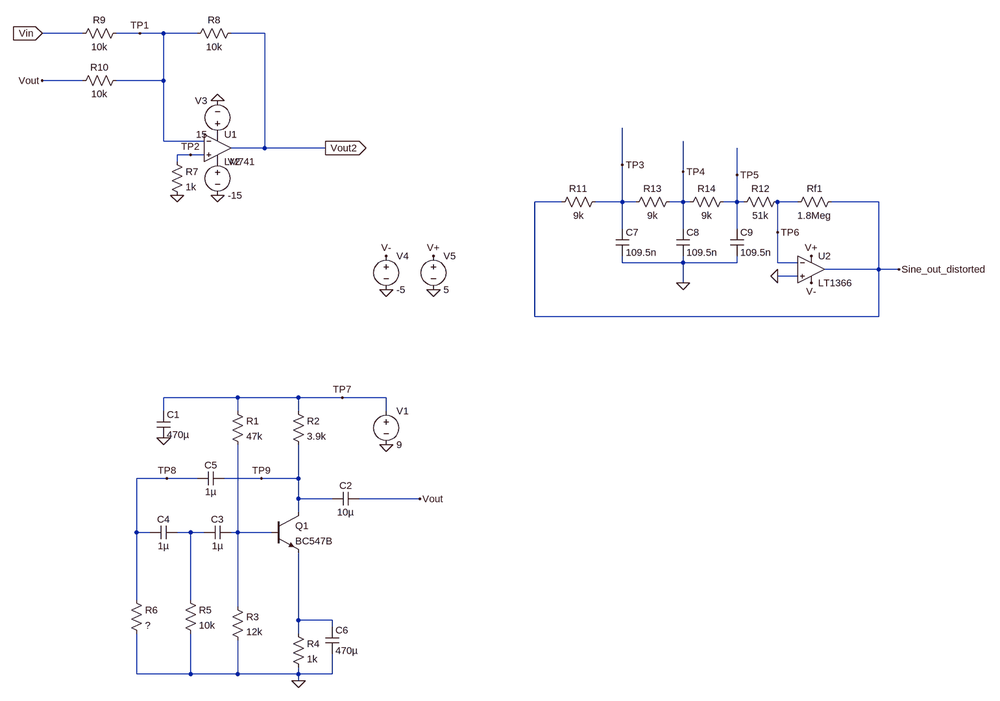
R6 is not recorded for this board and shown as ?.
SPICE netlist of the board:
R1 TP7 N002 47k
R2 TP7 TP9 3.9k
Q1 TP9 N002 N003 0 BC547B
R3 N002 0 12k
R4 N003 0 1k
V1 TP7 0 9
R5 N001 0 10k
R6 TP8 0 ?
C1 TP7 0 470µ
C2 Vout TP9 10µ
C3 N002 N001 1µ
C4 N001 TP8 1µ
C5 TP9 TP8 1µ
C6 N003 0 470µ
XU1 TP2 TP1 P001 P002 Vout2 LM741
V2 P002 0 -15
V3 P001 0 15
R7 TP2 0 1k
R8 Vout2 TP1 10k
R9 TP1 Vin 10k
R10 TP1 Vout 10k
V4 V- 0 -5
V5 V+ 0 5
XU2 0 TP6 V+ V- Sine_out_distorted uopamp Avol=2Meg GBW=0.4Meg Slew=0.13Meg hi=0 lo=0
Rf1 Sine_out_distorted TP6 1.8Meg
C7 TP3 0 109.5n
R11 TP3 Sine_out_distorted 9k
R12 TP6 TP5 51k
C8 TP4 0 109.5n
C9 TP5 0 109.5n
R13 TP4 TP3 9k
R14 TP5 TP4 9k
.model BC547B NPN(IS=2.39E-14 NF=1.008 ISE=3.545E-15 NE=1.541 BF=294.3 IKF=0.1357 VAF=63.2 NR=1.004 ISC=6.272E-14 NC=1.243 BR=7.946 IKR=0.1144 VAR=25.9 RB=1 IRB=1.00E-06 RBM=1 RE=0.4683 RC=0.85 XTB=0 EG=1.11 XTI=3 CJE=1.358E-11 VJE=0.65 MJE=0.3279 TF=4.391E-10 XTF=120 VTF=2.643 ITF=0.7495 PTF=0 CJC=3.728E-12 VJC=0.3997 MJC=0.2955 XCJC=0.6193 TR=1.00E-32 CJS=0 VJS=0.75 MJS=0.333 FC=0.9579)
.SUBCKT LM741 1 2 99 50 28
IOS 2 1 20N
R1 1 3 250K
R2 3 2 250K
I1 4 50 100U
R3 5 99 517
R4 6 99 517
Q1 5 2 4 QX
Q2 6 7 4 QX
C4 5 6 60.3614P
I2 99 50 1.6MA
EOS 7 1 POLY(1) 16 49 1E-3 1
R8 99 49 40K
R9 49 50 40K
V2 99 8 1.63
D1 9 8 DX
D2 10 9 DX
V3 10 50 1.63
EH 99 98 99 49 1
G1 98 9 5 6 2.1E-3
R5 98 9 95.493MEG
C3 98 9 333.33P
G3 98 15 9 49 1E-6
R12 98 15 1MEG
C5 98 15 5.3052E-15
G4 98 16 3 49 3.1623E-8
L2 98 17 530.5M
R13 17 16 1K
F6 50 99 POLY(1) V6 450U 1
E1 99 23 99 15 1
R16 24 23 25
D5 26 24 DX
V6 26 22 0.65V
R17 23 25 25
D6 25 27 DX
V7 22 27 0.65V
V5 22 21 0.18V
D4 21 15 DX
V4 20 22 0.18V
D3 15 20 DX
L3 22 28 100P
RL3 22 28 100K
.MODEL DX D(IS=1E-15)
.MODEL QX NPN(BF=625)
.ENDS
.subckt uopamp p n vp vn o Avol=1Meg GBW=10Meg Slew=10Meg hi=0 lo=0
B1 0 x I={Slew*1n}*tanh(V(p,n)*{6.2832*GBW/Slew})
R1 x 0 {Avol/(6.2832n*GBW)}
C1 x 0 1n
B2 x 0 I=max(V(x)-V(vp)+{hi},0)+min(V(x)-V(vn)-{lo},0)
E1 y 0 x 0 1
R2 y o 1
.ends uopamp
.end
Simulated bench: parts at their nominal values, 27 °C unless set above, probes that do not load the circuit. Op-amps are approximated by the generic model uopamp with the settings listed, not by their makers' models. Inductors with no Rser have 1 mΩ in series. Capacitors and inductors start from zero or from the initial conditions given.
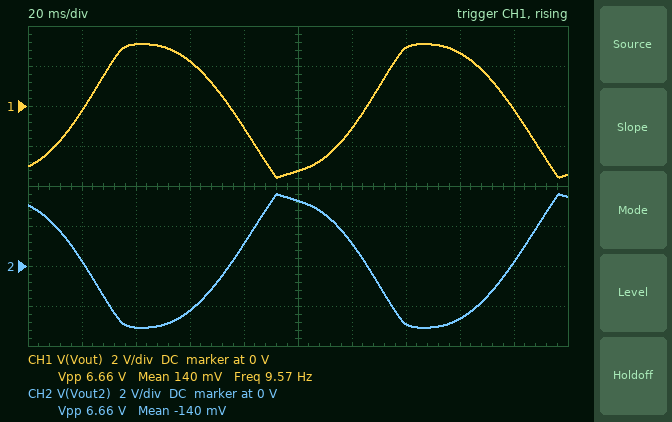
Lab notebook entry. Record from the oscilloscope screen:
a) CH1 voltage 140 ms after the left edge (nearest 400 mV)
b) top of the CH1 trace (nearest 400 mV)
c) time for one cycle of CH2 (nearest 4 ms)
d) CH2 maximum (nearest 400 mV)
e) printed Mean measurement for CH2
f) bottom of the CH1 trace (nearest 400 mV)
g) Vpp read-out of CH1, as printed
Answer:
2.8 V
3.2 V
104 ms
3.6 V
-140 mV
-3.6 V
6.66 V
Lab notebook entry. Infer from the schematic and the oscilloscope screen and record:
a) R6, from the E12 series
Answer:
5.6 kΩ
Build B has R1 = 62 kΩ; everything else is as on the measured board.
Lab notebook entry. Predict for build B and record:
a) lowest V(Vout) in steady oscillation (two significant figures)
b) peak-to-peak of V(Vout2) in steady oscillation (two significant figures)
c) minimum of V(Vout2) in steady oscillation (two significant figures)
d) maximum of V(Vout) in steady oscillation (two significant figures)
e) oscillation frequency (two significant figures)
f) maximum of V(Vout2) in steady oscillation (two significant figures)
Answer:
-2.5 V
4.8 V
-2.3 V
2.3 V
8.6 Hz
2.5 V
